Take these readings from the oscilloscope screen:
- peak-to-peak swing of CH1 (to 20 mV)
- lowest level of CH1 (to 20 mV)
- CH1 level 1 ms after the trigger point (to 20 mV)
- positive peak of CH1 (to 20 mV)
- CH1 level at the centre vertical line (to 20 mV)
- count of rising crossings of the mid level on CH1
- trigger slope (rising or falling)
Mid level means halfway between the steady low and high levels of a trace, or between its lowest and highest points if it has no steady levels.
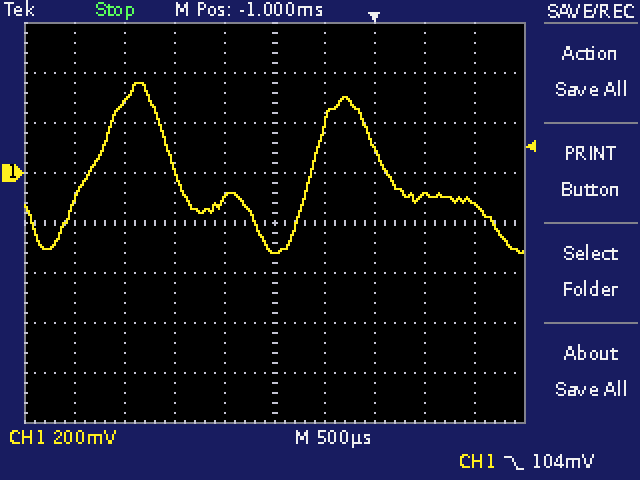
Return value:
680 mV
-320 mV
-120 mV
360 mV
-320 mV
2
falling
